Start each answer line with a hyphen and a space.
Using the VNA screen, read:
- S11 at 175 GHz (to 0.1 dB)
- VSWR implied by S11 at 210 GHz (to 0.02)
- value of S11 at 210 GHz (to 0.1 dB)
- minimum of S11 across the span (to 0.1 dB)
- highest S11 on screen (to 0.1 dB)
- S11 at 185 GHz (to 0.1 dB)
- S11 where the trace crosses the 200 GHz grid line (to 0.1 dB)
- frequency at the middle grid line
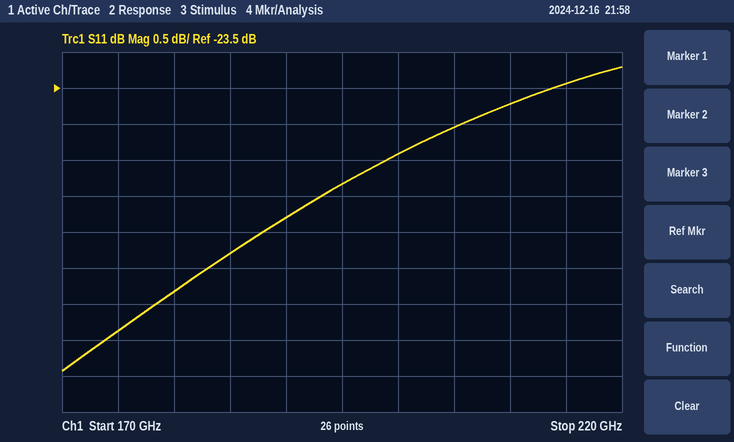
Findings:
- -26.9 dB
- 1.14
- -23.7 dB
- -27.4 dB
- -23.2 dB
- -25.8 dB
- -24.4 dB
- 195 GHz
